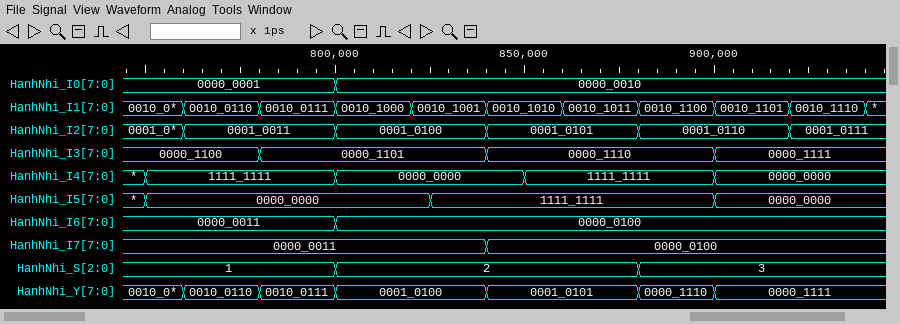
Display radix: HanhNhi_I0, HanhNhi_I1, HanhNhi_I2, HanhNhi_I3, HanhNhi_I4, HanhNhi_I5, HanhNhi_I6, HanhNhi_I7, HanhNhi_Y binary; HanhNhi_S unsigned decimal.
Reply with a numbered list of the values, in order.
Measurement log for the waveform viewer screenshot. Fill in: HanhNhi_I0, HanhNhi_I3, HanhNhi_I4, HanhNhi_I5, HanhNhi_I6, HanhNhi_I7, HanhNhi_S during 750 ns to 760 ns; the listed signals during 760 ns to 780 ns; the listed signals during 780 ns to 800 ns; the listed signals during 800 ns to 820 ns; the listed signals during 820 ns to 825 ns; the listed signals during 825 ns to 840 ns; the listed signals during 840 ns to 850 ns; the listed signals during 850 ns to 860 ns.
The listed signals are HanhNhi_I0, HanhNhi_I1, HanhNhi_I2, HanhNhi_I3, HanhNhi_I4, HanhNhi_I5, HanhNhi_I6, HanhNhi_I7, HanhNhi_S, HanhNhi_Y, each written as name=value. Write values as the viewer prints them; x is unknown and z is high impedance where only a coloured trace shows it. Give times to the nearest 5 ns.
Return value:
1. HanhNhi_I0=0000_0001, HanhNhi_I3=0000_1100, HanhNhi_I4=1111_1111, HanhNhi_I5=0000_0000, HanhNhi_I6=0000_0011, HanhNhi_I7=0000_0011, HanhNhi_S=1
2. HanhNhi_I0=0000_0001, HanhNhi_I1=0010_0110, HanhNhi_I2=0001_0011, HanhNhi_I3=0000_1100, HanhNhi_I4=1111_1111, HanhNhi_I5=0000_0000, HanhNhi_I6=0000_0011, HanhNhi_I7=0000_0011, HanhNhi_S=1, HanhNhi_Y=0010_0110
3. HanhNhi_I0=0000_0001, HanhNhi_I1=0010_0111, HanhNhi_I2=0001_0011, HanhNhi_I3=0000_1101, HanhNhi_I4=1111_1111, HanhNhi_I5=0000_0000, HanhNhi_I6=0000_0011, HanhNhi_I7=0000_0011, HanhNhi_S=1, HanhNhi_Y=0010_0111
4. HanhNhi_I0=0000_0010, HanhNhi_I1=0010_1000, HanhNhi_I2=0001_0100, HanhNhi_I3=0000_1101, HanhNhi_I4=0000_0000, HanhNhi_I5=0000_0000, HanhNhi_I6=0000_0100, HanhNhi_I7=0000_0011, HanhNhi_S=2, HanhNhi_Y=0001_0100
5. HanhNhi_I0=0000_0010, HanhNhi_I1=0010_1001, HanhNhi_I2=0001_0100, HanhNhi_I3=0000_1101, HanhNhi_I4=0000_0000, HanhNhi_I5=0000_0000, HanhNhi_I6=0000_0100, HanhNhi_I7=0000_0011, HanhNhi_S=2, HanhNhi_Y=0001_0100
6. HanhNhi_I0=0000_0010, HanhNhi_I1=0010_1001, HanhNhi_I2=0001_0100, HanhNhi_I3=0000_1101, HanhNhi_I4=0000_0000, HanhNhi_I5=1111_1111, HanhNhi_I6=0000_0100, HanhNhi_I7=0000_0011, HanhNhi_S=2, HanhNhi_Y=0001_0100
7. HanhNhi_I0=0000_0010, HanhNhi_I1=0010_1010, HanhNhi_I2=0001_0101, HanhNhi_I3=0000_1110, HanhNhi_I4=0000_0000, HanhNhi_I5=1111_1111, HanhNhi_I6=0000_0100, HanhNhi_I7=0000_0100, HanhNhi_S=2, HanhNhi_Y=0001_0101
8. HanhNhi_I0=0000_0010, HanhNhi_I1=0010_1010, HanhNhi_I2=0001_0101, HanhNhi_I3=0000_1110, HanhNhi_I4=1111_1111, HanhNhi_I5=1111_1111, HanhNhi_I6=0000_0100, HanhNhi_I7=0000_0100, HanhNhi_S=2, HanhNhi_Y=0001_0101
